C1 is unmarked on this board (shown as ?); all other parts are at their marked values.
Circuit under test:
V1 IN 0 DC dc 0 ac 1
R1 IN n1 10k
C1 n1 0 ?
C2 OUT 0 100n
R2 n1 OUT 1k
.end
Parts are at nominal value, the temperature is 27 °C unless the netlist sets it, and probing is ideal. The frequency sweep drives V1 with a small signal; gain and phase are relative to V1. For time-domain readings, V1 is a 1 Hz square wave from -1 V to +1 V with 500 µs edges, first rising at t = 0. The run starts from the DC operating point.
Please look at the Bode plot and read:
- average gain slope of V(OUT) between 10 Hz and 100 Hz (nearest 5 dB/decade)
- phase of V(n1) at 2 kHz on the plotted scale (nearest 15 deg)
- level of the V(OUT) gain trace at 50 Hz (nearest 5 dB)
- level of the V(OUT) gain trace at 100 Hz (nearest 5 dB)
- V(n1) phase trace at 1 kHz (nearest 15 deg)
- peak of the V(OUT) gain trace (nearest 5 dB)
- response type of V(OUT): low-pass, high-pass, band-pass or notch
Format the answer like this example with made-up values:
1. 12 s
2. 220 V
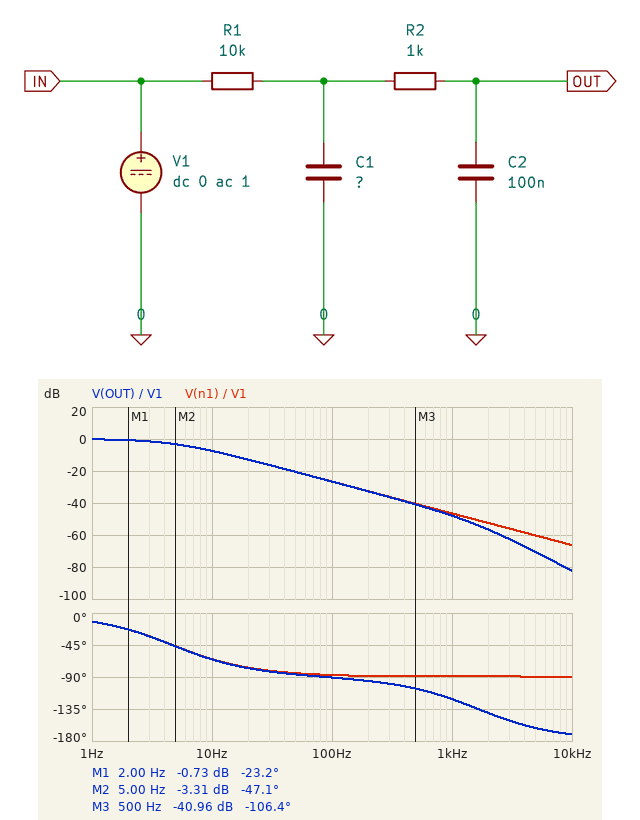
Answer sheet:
1. -20 dB/decade
2. -90 deg
3. -20 dB
4. -25 dB
5. -90 deg
6. 0 dB
7. low-pass
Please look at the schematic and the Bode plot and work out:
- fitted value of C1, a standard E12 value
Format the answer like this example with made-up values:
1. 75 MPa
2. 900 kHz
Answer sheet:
1. 3.3 µF
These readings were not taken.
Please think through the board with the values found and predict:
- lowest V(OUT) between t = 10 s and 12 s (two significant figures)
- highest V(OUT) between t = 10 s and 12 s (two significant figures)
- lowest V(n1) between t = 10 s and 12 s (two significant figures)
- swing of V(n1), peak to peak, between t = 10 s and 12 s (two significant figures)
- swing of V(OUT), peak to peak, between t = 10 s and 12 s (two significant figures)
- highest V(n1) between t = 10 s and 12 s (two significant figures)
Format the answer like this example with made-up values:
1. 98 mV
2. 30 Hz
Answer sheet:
1. -1.0 V
2. 1.0 V
3. -1.0 V
4. 2.0 V
5. 2.0 V
6. 1.0 V
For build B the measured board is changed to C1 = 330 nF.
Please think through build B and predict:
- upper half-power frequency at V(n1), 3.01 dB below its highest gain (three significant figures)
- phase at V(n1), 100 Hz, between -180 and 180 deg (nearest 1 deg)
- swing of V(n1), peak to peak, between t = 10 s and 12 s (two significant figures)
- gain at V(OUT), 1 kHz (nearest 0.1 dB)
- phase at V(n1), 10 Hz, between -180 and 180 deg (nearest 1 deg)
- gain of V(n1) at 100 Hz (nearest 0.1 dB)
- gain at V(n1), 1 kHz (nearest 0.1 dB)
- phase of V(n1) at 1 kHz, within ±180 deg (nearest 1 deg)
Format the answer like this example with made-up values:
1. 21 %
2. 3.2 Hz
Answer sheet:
1. 36.8 Hz
2. -69 deg
3. 2.0 V
4. -29.6 dB
5. -15 deg
6. -9.2 dB
7. -28.1 dB
8. -81 deg
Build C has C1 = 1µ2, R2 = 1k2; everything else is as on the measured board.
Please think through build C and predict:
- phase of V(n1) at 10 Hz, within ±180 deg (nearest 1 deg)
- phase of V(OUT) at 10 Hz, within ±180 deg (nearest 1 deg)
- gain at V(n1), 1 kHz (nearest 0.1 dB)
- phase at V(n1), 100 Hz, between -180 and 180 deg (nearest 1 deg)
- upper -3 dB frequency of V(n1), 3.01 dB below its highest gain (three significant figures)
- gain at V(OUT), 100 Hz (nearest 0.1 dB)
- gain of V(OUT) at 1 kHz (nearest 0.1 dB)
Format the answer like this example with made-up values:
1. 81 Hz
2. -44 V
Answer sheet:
1. -39 deg
2. -40 deg
3. -38.0 dB
4. -83 deg
5. 12.2 Hz
6. -18.3 dB
7. -40.0 dB
